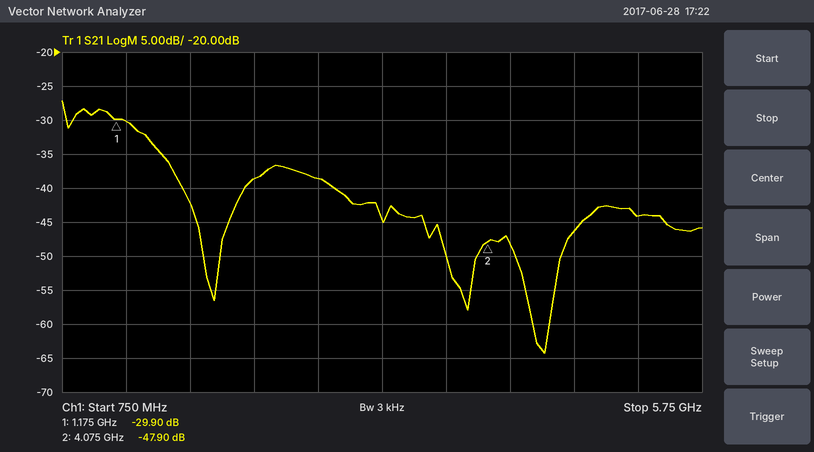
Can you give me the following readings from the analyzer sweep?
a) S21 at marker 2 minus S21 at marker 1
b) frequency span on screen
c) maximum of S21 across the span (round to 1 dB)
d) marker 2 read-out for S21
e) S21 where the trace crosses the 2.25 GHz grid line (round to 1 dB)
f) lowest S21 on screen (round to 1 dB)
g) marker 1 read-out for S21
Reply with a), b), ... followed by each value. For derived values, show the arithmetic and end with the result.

a) -47.9 − (-29.9) = -18.00 dB
b) 5 GHz
c) -27 dB
d) -47.90 dB
e) -39 dB
f) -64 dB
g) -29.90 dB
